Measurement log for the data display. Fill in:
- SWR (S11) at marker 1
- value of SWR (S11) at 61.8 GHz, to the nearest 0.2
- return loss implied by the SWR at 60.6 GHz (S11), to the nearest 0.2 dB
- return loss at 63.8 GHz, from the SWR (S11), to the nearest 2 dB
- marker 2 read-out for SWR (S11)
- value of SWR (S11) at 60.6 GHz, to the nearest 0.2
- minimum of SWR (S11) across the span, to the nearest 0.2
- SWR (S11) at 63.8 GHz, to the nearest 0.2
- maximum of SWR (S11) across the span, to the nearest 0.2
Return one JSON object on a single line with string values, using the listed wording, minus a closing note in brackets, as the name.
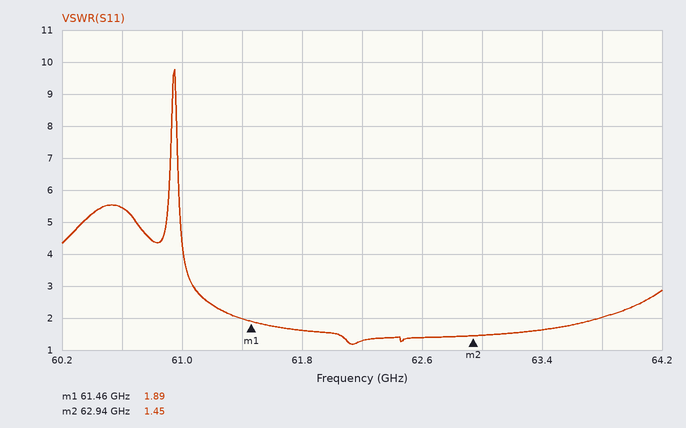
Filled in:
{"SWR (S11) at marker 1": "1.89", "value of SWR (S11) at 61.8 GHz, to the nearest 0.2": "1.6", "return loss implied by the SWR at 60.6 GHz (S11), to the nearest 0.2 dB": "3.2 dB", "return loss at 63.8 GHz, from the SWR (S11), to the nearest 2 dB": "10 dB", "marker 2 read-out for SWR": "1.45", "value of SWR (S11) at 60.6 GHz, to the nearest 0.2": "5.4", "minimum of SWR (S11) across the span, to the nearest 0.2": "1.2", "SWR (S11) at 63.8 GHz, to the nearest 0.2": "2.0", "maximum of SWR (S11) across the span, to the nearest 0.2": "9.8"}
